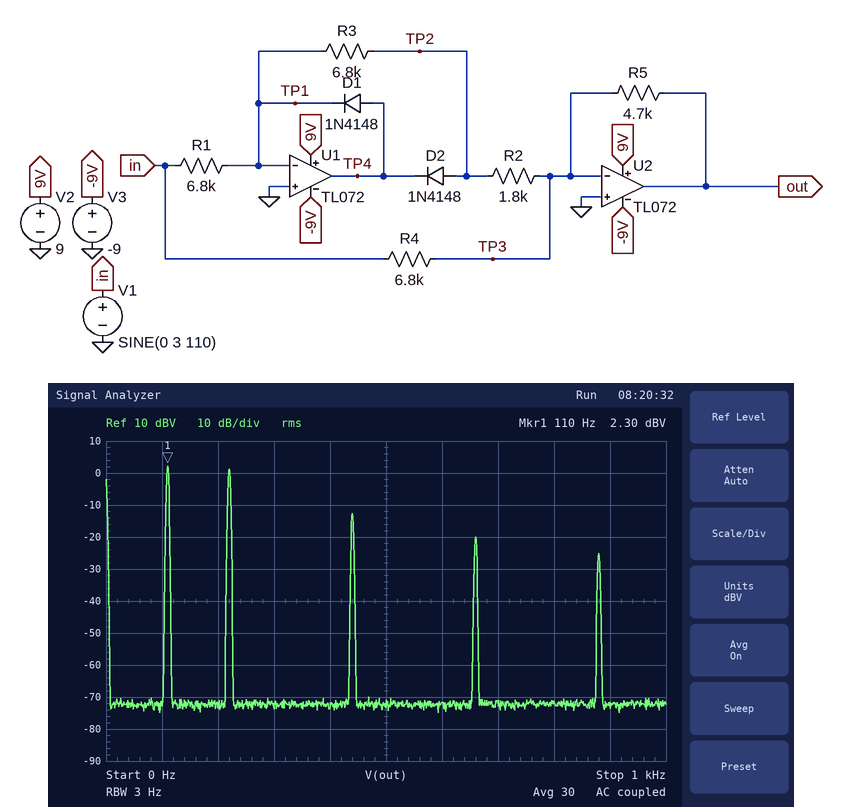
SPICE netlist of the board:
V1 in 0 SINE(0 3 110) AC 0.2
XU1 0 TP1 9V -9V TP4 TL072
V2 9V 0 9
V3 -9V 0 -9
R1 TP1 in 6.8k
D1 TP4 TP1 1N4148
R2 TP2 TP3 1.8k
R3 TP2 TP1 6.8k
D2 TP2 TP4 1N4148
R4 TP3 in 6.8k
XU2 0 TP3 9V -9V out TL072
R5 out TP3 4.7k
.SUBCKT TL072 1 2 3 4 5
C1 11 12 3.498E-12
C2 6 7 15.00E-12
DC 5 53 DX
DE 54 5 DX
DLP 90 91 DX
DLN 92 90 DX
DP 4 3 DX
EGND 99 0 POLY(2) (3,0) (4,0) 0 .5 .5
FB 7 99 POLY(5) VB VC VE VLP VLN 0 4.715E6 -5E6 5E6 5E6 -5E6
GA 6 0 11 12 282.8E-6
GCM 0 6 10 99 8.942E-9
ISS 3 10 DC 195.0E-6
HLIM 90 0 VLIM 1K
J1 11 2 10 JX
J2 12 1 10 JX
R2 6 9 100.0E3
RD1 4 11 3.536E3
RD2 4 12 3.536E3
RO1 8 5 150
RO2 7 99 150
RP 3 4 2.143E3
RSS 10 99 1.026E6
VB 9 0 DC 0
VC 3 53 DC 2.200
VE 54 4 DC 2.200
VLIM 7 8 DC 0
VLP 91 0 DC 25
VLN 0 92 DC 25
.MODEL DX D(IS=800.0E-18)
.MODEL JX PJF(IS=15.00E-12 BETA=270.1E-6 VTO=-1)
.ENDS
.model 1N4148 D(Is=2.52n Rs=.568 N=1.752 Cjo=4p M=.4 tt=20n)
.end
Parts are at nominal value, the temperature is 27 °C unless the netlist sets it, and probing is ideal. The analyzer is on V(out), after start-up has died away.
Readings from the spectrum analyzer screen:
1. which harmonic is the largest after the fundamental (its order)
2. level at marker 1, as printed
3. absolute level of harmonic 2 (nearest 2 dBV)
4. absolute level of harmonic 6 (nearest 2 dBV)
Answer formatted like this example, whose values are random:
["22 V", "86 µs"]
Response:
["2", "2.30 dBV", "2 dBV", "-20 dBV"]
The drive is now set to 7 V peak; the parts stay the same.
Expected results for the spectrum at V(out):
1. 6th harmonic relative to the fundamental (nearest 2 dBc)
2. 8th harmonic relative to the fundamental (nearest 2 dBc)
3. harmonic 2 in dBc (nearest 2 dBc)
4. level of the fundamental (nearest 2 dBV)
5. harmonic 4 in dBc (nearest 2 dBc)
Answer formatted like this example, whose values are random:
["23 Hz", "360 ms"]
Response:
["-12 dBc", "-20 dBc", "0 dBc", "4 dBV", "-6 dBc"]
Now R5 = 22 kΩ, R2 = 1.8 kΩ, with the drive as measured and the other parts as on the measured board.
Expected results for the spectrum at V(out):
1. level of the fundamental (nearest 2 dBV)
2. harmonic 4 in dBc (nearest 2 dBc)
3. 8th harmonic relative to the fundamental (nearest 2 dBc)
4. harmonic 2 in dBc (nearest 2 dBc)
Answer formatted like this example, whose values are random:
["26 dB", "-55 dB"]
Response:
["-10 dBV", "8 dBc", "0 dBc", "14 dBc"]
